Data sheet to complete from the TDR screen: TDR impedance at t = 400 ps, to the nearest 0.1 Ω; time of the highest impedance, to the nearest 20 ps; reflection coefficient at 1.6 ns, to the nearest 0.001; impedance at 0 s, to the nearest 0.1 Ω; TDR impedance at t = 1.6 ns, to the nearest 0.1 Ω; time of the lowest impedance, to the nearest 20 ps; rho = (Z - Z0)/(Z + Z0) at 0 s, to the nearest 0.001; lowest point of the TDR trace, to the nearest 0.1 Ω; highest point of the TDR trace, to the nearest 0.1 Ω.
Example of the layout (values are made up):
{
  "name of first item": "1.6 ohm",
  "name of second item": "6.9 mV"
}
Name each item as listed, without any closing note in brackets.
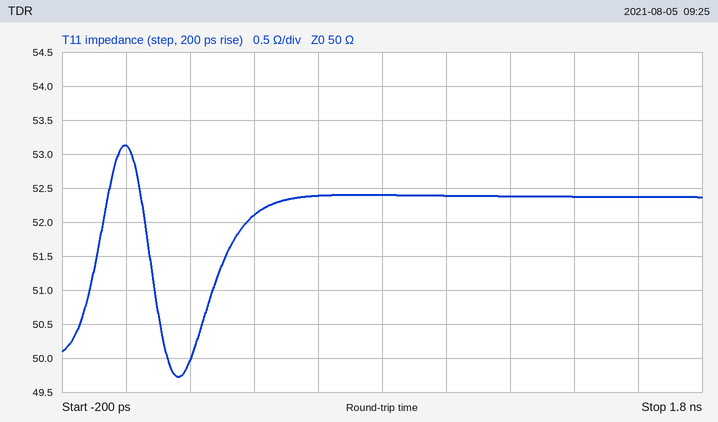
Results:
{
  "TDR impedance at t = 400 ps, to the nearest 0.1 Ω": "52.1 Ω",
  "time of the highest impedance, to the nearest 20 ps": "0 ps",
  "reflection coefficient at 1.6 ns, to the nearest 0.001": "+0.023",
  "impedance at 0 s, to the nearest 0.1 Ω": "53.1 Ω",
  "TDR impedance at t = 1.6 ns, to the nearest 0.1 Ω": "52.4 Ω",
  "time of the lowest impedance, to the nearest 20 ps": "160 ps",
  "rho = (Z - Z0)/(Z + Z0) at 0 s, to the nearest 0.001": "+0.030",
  "lowest point of the TDR trace, to the nearest 0.1 Ω": "49.7 Ω",
  "highest point of the TDR trace, to the nearest 0.1 Ω": "53.1 Ω"
}
